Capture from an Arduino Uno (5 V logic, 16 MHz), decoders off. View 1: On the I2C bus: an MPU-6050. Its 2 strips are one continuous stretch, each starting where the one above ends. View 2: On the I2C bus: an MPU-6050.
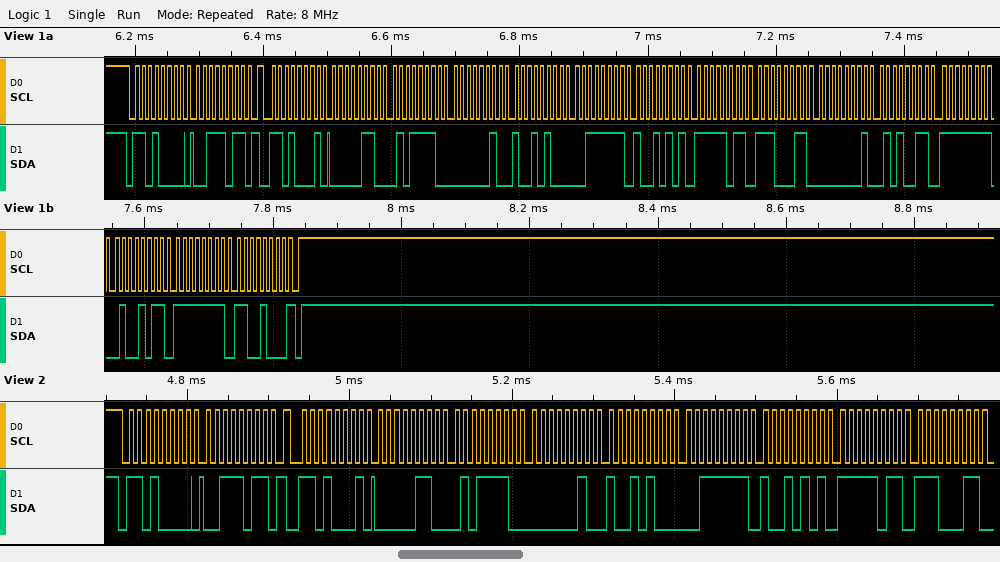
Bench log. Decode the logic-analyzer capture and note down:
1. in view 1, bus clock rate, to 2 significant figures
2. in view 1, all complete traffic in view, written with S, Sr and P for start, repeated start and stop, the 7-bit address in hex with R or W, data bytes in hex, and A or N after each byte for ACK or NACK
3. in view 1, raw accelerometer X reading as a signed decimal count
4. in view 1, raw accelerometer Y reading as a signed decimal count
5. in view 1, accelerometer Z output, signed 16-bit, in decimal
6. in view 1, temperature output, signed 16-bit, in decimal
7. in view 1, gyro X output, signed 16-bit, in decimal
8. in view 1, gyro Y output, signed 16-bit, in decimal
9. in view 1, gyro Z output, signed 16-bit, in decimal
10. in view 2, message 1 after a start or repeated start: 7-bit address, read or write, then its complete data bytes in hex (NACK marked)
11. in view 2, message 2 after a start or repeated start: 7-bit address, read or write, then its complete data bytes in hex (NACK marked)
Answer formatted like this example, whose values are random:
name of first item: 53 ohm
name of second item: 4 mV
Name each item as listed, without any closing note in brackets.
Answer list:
in view 1, bus clock rate, to 2 significant figures: 100 kHz
in view 1, all complete traffic in view, written with S, Sr and P for start, repeated start and stop, the 7-bit address in hex with R or W, data bytes in hex, and A or N after each byte for ACK or NACK: S 68W A 3B A Sr 68R A 06 A 5E A 02 A 94 A 3F A 95 A FB A E3 A 01 A 53 A FF A 4B A FF A C8 N P
in view 1, raw accelerometer X reading as a signed decimal count: 1630
in view 1, raw accelerometer Y reading as a signed decimal count: 660
in view 1, accelerometer Z output, signed 16-bit, in decimal: 16277
in view 1, temperature output, signed 16-bit, in decimal: -1053
in view 1, gyro X output, signed 16-bit, in decimal: 339
in view 1, gyro Y output, signed 16-bit, in decimal: -181
in view 1, gyro Z output, signed 16-bit, in decimal: -56
in view 2, message 1 after a start or repeated start: 7-bit address, read or write, then its complete data bytes in hex: 0x68 write: 3B
in view 2, message 2 after a start or repeated start: 7-bit address, read or write, then its complete data bytes in hex: 0x68 read: 06 5E 02 94 3F 95 FB E3
